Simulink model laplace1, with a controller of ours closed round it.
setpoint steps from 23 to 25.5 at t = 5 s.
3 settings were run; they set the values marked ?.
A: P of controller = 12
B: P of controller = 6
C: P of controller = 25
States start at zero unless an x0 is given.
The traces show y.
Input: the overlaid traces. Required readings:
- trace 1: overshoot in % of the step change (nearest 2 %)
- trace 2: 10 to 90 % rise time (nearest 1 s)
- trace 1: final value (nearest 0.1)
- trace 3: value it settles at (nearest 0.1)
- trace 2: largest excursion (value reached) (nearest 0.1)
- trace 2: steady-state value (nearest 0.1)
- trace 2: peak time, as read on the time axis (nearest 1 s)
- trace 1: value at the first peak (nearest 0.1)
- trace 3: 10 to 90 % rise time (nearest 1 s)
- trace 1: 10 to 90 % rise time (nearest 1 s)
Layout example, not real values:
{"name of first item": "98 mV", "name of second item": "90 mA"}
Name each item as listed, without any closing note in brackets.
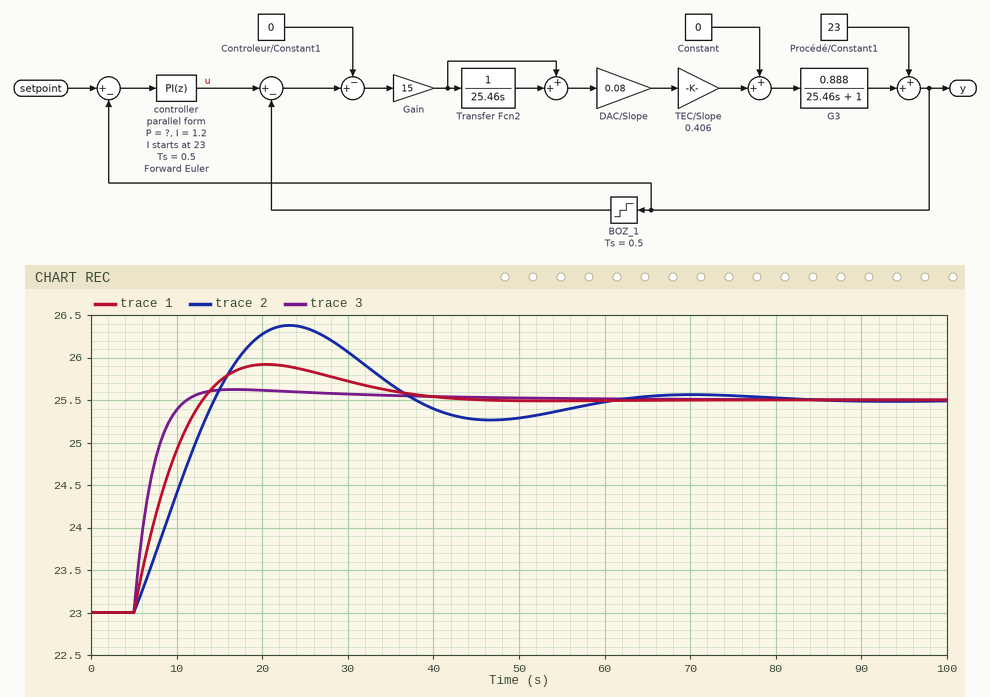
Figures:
{"trace 1: overshoot in % of the step change": "16 %", "trace 2: 10 to 90 % rise time": "7 s", "trace 1: final value": "25.5", "trace 3: value it settles at": "25.5", "trace 2: largest excursion (value reached)": "26.4", "trace 2: steady-state value": "25.5", "trace 2: peak time, as read on the time axis": "23 s", "trace 1: value at the first peak": "25.9", "trace 3: 10 to 90 % rise time": "4 s", "trace 1: 10 to 90 % rise time": "6 s"}
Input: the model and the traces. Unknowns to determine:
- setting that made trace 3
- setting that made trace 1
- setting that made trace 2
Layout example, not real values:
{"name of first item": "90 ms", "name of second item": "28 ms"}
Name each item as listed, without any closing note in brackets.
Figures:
{"setting that made trace 3": "C", "setting that made trace 1": "A", "setting that made trace 2": "B"}
